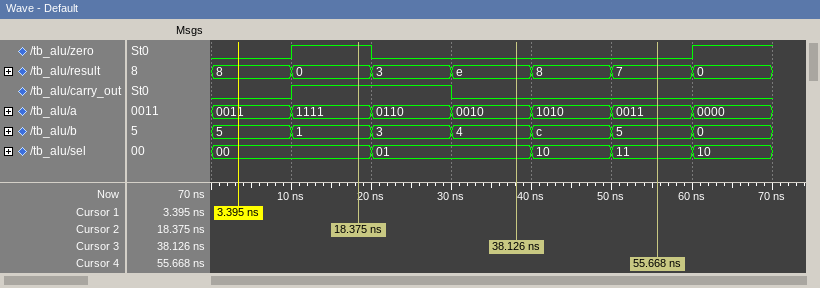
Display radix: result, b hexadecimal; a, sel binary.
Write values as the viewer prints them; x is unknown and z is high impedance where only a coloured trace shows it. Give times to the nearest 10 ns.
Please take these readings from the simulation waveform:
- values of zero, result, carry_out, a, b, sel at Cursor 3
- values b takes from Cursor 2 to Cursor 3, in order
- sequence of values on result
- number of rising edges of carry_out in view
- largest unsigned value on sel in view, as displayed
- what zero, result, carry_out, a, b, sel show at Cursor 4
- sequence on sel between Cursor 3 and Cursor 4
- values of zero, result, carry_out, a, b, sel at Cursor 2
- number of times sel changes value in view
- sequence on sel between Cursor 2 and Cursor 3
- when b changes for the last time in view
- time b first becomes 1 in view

zero=0, result=e, carry_out=0, a=0010, b=4, sel=01
1, 3, 4
8, 0, 3, e, 8, 7, 0
1
11
zero=0, result=7, carry_out=0, a=0011, b=5, sel=11
01, 10, 11
zero=1, result=0, carry_out=1, a=1111, b=1, sel=00
4
00, 01
60 ns
10 ns
